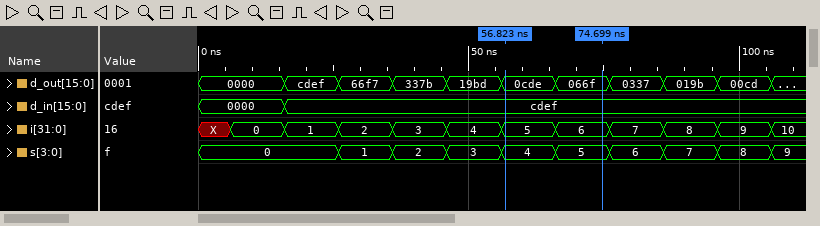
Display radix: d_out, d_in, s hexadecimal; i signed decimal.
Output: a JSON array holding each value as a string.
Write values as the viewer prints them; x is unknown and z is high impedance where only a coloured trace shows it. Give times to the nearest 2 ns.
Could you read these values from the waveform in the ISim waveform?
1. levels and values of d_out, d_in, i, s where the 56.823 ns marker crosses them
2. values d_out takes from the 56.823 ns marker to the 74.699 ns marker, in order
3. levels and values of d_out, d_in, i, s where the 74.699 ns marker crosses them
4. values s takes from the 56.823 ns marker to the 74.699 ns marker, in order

["d_out=0cde, d_in=cdef, i=5, s=4", "0cde, 066f", "d_out=066f, d_in=cdef, i=6, s=5", "4, 5"]
